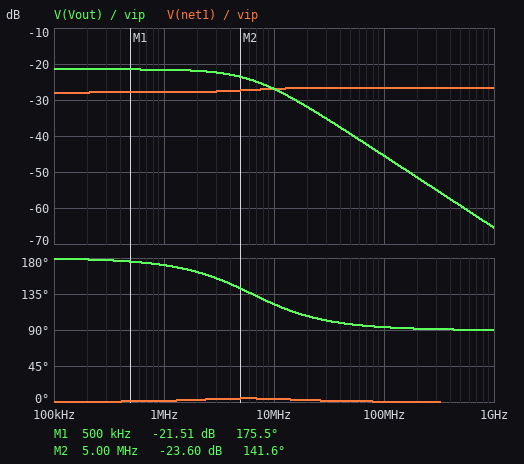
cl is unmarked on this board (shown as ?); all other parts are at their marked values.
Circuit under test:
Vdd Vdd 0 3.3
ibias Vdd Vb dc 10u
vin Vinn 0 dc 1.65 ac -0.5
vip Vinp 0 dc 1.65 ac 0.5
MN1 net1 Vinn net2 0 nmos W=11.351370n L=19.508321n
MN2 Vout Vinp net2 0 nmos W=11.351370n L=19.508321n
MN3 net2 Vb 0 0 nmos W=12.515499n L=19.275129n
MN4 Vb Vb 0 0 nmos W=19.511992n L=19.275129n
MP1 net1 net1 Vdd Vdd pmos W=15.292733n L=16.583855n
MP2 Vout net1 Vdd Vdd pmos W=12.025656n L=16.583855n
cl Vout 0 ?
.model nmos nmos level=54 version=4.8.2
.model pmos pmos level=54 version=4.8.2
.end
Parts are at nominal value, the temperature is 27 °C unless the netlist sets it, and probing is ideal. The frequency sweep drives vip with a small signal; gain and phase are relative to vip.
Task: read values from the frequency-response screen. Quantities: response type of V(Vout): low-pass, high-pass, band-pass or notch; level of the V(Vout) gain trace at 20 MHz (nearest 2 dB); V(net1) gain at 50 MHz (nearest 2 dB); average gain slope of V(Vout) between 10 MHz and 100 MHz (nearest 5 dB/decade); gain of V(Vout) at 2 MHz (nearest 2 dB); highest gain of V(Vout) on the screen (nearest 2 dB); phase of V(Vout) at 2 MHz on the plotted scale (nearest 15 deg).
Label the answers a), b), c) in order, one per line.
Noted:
a) low-pass
b) -32 dB
c) -26 dB
d) -20 dB/decade
e) -22 dB
f) -22 dB
g) 165 deg
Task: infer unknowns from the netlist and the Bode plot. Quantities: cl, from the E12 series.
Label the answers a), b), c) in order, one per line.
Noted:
a) 3.3 pF
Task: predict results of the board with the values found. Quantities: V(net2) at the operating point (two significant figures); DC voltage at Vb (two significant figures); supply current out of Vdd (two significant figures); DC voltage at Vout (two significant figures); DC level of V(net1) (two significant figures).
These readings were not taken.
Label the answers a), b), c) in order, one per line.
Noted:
a) 2.2 V
b) 50 mV
c) 150 µA
d) 2.7 V
e) 2.7 V
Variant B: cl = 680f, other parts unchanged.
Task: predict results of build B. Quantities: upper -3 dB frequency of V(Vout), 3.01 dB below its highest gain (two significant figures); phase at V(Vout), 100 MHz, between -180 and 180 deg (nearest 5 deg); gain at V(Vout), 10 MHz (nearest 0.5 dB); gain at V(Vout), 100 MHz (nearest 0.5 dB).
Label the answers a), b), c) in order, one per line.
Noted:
a) 31 MHz
b) 105 deg
c) -22.0 dB
d) -32.0 dB
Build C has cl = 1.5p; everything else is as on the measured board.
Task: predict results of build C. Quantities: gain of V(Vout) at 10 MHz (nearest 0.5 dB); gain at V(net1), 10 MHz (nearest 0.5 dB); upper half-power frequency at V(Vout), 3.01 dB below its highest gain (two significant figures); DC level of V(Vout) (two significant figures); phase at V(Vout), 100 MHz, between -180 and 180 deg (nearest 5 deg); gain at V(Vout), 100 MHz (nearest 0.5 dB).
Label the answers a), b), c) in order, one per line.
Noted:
a) -23.5 dB
b) -27.5 dB
c) 14 MHz
d) 2.7 V
e) 100 deg
f) -38.5 dB
